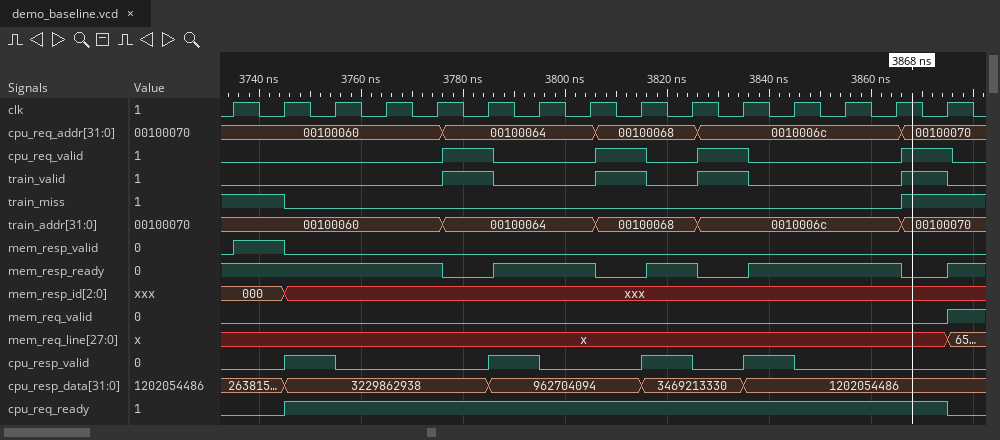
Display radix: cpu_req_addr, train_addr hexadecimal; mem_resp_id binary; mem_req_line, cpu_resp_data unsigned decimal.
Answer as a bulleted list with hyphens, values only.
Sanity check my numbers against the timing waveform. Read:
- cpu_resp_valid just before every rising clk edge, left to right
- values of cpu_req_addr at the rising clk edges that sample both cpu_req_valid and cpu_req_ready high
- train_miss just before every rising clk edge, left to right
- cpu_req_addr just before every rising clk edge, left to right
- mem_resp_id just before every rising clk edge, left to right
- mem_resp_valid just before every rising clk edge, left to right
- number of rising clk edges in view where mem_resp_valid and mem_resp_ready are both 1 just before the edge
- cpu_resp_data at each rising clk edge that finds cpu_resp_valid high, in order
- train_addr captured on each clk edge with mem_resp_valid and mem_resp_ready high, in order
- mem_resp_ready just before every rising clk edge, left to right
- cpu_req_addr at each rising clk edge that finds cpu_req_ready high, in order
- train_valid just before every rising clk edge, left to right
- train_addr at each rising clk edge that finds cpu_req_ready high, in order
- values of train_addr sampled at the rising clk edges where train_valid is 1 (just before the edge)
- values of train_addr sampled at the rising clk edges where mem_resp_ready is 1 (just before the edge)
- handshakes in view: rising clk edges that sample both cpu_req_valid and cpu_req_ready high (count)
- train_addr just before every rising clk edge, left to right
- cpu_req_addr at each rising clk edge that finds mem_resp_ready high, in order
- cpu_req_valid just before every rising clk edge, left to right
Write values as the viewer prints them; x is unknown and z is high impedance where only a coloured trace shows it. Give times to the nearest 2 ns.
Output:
- 0 0 1 0 0 0 1 0 0 1 0 1 0 0 0
- 00100064, 00100068, 0010006c, 00100070
- 1 1 0 0 0 0 0 0 0 0 0 0 0 0 1
- 00100060, 00100060, 00100060, 00100060, 00100060, 00100064, 00100064, 00100064, 00100068, 00100068, 0010006c, 0010006c, 0010006c, 0010006c, 00100070
- 000, 000, xxx, xxx, xxx, xxx, xxx, xxx, xxx, xxx, xxx, xxx, xxx, xxx, xxx
- 0 1 0 0 0 0 0 0 0 0 0 0 0 0 0
- 1
- 3229862938, 962704094, 3469213330, 1202054486
- 00100060
- 1 1 1 1 1 0 1 1 0 1 0 1 1 1 0
- 00100060, 00100060, 00100060, 00100064, 00100064, 00100064, 00100068, 00100068, 0010006c, 0010006c, 0010006c, 0010006c, 00100070
- 0 0 0 0 0 1 0 0 1 0 1 0 0 0 1
- 00100060, 00100060, 00100060, 00100064, 00100064, 00100064, 00100068, 00100068, 0010006c, 0010006c, 0010006c, 0010006c, 00100070
- 00100064, 00100068, 0010006c, 00100070
- 00100060, 00100060, 00100060, 00100060, 00100060, 00100064, 00100064, 00100068, 0010006c, 0010006c, 0010006c
- 4
- 00100060, 00100060, 00100060, 00100060, 00100060, 00100064, 00100064, 00100064, 00100068, 00100068, 0010006c, 0010006c, 0010006c, 0010006c, 00100070
- 00100060, 00100060, 00100060, 00100060, 00100060, 00100064, 00100064, 00100068, 0010006c, 0010006c, 0010006c
- 0 0 0 0 0 1 0 0 1 0 1 0 0 0 1
